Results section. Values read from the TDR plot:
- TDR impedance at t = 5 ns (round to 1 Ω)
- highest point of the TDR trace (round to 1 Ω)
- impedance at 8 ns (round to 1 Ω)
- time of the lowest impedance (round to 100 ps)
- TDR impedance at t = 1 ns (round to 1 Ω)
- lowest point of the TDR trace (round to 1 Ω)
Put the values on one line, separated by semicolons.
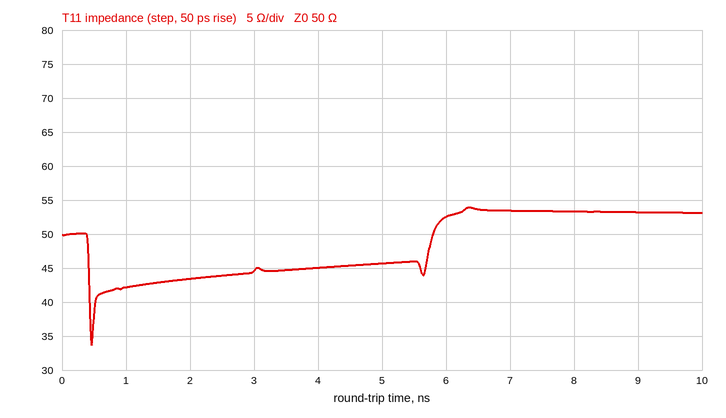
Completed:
46 Ω; 54 Ω; 53 Ω; 500 ps; 42 Ω; 34 Ω
